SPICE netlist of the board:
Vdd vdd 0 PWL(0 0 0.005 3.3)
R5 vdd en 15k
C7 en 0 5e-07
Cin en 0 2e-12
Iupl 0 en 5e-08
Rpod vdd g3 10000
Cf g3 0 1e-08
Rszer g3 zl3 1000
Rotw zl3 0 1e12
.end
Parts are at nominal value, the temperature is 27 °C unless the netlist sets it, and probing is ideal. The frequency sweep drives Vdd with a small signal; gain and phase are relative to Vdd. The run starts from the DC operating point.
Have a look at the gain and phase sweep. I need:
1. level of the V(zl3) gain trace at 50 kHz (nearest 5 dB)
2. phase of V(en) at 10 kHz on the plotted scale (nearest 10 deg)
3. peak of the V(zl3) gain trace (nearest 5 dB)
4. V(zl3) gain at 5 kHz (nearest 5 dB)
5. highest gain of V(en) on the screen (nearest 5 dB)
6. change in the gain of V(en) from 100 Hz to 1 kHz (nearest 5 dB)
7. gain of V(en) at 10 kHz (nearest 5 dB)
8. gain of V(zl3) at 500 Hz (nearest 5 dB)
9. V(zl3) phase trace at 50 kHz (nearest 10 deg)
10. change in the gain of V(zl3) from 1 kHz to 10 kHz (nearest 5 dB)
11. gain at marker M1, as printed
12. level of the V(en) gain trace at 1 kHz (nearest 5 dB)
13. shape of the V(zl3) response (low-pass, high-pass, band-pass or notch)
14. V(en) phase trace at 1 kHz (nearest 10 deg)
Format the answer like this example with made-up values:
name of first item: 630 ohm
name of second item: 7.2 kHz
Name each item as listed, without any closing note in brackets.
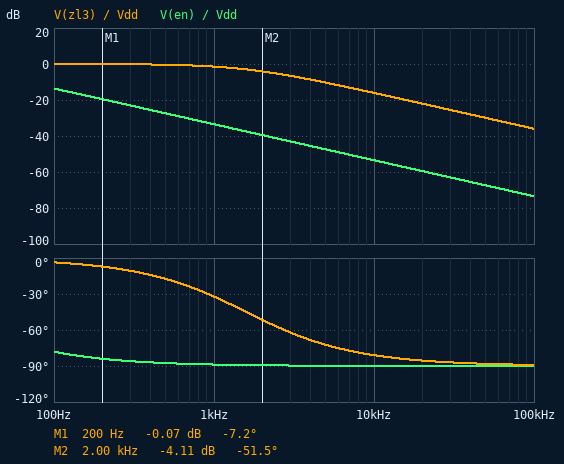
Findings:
level of the V(zl3) gain trace at 50 kHz: -30 dB
phase of V(en) at 10 kHz on the plotted scale: -90 deg
peak of the V(zl3) gain trace: 0 dB
V(zl3) gain at 5 kHz: -10 dB
highest gain of V(en) on the screen: -15 dB
change in the gain of V(en) from 100 Hz to 1 kHz: -20 dB
gain of V(en) at 10 kHz: -55 dB
gain of V(zl3) at 500 Hz: 0 dB
V(zl3) phase trace at 50 kHz: -90 deg
change in the gain of V(zl3) from 1 kHz to 10 kHz: -15 dB
gain at marker M1, as printed: -0.07 dB
level of the V(en) gain trace at 1 kHz: -35 dB
shape of the V(zl3) response: low-pass
V(en) phase trace at 1 kHz: -90 deg
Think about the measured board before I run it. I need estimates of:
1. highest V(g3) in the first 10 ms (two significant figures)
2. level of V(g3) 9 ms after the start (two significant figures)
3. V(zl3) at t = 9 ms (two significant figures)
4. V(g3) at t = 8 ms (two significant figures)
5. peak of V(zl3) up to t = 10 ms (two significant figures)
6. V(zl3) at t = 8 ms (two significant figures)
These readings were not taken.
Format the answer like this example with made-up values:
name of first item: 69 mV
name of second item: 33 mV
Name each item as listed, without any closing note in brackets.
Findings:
highest V(g3) in the first 10 ms: 3.3 V
level of V(g3) 9 ms after the start: 3.3 V
V(zl3) at t = 9 ms: 3.3 V
V(g3) at t = 8 ms: 3.3 V
peak of V(zl3) up to t = 10 ms: 3.3 V
V(zl3) at t = 8 ms: 3.3 V
